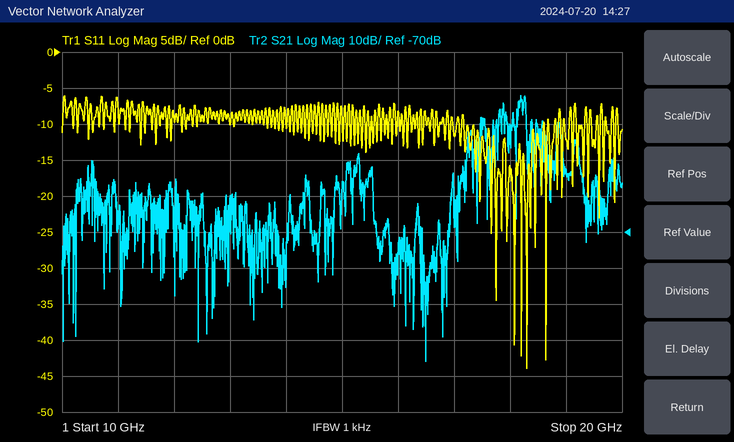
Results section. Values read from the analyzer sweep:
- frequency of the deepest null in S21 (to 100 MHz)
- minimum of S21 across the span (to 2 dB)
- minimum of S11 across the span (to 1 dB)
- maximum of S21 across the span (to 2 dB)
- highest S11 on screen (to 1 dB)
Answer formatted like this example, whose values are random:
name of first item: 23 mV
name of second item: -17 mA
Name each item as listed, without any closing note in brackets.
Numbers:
frequency of the deepest null in S21: 16.5 GHz
minimum of S21 across the span: -106 dB
minimum of S11 across the span: -44 dB
maximum of S21 across the span: -32 dB
highest S11 on screen: -6 dB
